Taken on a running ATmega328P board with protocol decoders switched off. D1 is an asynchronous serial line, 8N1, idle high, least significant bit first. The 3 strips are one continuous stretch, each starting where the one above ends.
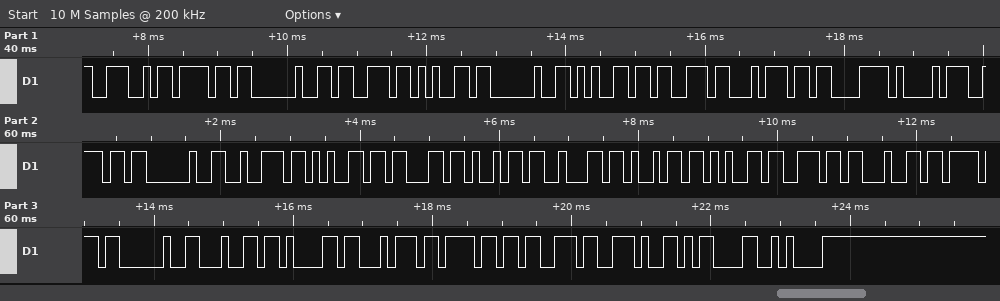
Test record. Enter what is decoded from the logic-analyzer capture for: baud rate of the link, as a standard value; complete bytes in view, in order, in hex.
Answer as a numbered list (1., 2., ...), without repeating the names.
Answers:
1. 9600 baud
2. 0x4E 0x6F 0x20 0x73 0x65 0x20 0x65 0x73 0x74 0xC3 0xA1 0x6E 0x20 0x72 0x65 0x63 0x69 0x62 0x69 0x65 0x6E 0x64 0x6F 0x20 0x64 0x61 0x74 0x6F 0x73 0x2E 0x0D 0x0A
